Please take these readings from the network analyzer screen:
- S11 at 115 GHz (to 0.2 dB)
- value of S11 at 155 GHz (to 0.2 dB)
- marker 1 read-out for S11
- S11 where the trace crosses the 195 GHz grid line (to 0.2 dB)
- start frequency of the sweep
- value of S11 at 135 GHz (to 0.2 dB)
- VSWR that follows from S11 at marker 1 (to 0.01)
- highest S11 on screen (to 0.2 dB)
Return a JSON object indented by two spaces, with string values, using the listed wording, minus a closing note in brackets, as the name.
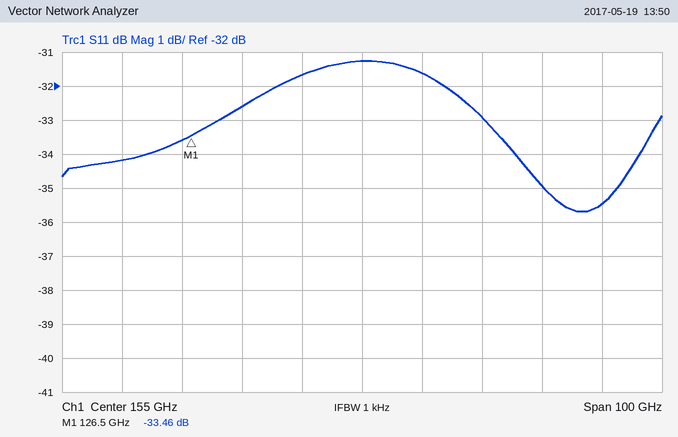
{
  "S11 at 115 GHz": "-34.2 dB",
  "value of S11 at 155 GHz": "-31.2 dB",
  "marker 1 read-out for S11": "-33.46 dB",
  "S11 where the trace crosses the 195 GHz grid line": "-35.4 dB",
  "start frequency of the sweep": "105 GHz",
  "value of S11 at 135 GHz": "-32.6 dB",
  "VSWR that follows from S11 at marker 1": "1.04",
  "highest S11 on screen": "-31.2 dB"
}
